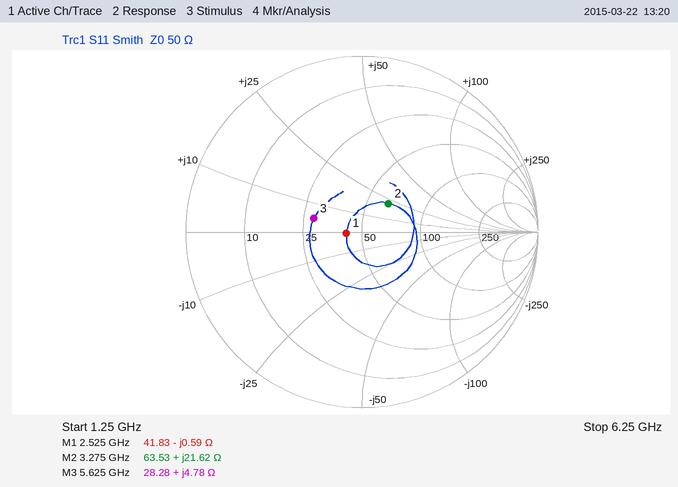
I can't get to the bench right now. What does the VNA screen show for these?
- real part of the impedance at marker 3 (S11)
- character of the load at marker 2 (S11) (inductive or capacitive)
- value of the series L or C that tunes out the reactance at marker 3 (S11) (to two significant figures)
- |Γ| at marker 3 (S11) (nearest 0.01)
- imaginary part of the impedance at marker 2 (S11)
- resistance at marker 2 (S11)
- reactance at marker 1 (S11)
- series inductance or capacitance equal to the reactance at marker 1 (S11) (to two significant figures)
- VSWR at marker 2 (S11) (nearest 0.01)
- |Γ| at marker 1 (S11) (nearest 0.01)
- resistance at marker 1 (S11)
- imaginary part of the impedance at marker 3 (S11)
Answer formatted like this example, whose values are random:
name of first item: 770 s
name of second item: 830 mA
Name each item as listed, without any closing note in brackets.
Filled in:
real part of the impedance at marker 3: 28.28 Ω
character of the load at marker 2 (S11): inductive
value of the series L or C that tunes out the reactance at marker 3 (S11): 5.9 pF
|Γ| at marker 3 (S11): 0.28
imaginary part of the impedance at marker 2: +21.62 Ω
resistance at marker 2: 63.53 Ω
reactance at marker 1: -0.59 Ω
series inductance or capacitance equal to the reactance at marker 1 (S11): 110 pF
VSWR at marker 2 (S11): 1.57
|Γ| at marker 1 (S11): 0.09
resistance at marker 1: 41.83 Ω
imaginary part of the impedance at marker 3: +4.78 Ω
